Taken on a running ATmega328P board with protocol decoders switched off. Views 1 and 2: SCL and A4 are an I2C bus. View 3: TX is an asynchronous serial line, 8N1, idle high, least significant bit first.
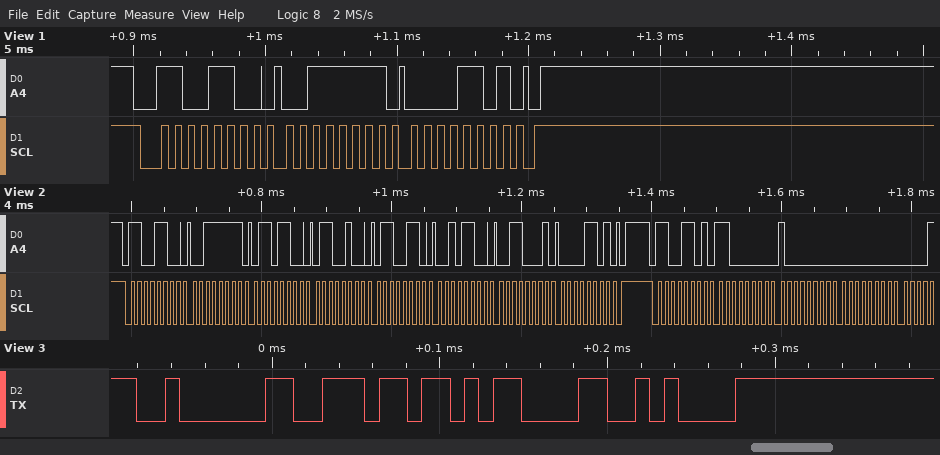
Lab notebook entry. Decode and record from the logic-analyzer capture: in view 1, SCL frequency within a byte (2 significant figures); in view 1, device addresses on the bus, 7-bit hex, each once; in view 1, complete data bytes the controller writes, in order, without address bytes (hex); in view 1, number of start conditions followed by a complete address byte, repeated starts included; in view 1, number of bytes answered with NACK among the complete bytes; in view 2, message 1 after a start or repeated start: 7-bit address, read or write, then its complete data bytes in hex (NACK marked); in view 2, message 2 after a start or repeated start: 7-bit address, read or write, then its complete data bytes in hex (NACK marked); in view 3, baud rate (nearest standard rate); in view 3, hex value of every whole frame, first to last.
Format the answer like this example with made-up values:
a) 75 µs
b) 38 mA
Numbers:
a) 100 kHz
b) 0x66
c) 3F 0D
d) 1
e) 0
f) 0x66 write: 3F 6C 64 66 2C 31 0D
g) 0x66 read: C0 80 00
h) 115200 baud
i) 02 6E 0D 0A
